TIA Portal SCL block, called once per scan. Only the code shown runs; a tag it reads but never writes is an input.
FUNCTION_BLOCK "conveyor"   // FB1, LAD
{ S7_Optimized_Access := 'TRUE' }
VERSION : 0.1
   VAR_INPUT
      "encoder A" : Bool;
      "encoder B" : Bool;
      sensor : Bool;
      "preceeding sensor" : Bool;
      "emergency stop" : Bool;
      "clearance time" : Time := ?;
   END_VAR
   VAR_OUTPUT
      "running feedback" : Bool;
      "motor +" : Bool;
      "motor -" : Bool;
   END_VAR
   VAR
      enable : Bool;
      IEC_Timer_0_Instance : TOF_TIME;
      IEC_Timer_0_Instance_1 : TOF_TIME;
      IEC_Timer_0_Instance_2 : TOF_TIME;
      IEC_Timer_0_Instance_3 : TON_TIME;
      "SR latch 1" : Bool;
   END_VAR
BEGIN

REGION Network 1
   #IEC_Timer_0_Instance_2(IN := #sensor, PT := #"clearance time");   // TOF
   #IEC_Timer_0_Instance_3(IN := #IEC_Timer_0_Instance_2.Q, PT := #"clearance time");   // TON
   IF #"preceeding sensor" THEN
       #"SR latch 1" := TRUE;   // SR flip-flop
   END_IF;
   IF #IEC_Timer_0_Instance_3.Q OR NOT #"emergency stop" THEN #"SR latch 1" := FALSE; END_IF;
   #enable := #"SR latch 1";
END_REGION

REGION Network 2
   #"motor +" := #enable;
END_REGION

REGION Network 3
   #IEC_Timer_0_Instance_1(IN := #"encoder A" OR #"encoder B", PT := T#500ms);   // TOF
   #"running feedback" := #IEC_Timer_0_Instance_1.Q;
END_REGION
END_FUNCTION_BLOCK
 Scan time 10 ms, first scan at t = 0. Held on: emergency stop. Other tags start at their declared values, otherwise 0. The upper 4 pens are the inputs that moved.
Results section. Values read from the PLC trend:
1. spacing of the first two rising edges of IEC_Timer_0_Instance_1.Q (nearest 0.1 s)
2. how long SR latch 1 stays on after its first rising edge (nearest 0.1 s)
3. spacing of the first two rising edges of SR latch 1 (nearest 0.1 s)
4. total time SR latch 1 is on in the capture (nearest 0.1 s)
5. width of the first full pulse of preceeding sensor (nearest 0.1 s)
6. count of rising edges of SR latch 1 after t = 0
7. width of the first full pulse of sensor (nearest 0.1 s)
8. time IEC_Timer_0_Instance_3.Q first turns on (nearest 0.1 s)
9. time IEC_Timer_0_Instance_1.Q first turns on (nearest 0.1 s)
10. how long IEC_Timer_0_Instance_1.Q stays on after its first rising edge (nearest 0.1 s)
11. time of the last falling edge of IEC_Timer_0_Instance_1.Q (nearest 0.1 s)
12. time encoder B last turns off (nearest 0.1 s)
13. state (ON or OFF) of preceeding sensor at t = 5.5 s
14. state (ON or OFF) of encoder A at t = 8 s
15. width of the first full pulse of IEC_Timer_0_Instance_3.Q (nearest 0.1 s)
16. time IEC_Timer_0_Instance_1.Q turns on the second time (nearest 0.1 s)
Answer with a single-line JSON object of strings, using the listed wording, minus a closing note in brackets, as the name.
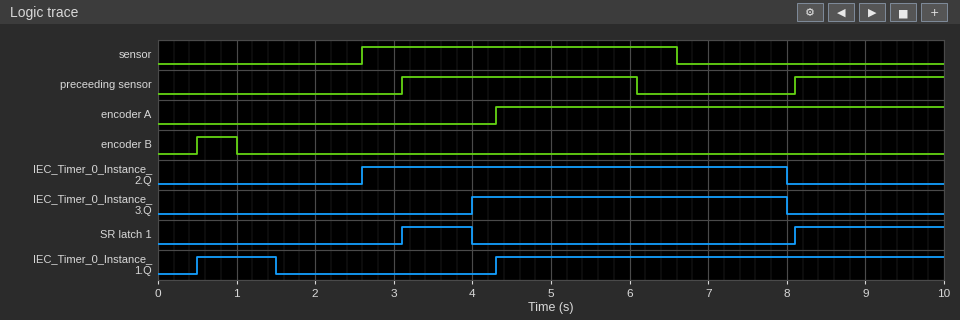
{"spacing of the first two rising edges of IEC_Timer_0_Instance_1.Q": "3.8 s", "how long SR latch 1 stays on after its first rising edge": "0.9 s", "spacing of the first two rising edges of SR latch 1": "5.0 s", "total time SR latch 1 is on in the capture": "2.8 s", "width of the first full pulse of preceeding sensor": "3.0 s", "count of rising edges of SR latch 1 after t = 0": "2", "width of the first full pulse of sensor": "4.0 s", "time IEC_Timer_0_Instance_3.Q first turns on": "4.0 s", "time IEC_Timer_0_Instance_1.Q first turns on": "0.5 s", "how long IEC_Timer_0_Instance_1.Q stays on after its first rising edge": "1.0 s", "time of the last falling edge of IEC_Timer_0_Instance_1.Q": "1.5 s", "time encoder B last turns off": "1.0 s", "state (ON or OFF) of preceeding sensor at t = 5.5 s": "ON", "state (ON or OFF) of encoder A at t = 8 s": "ON", "width of the first full pulse of IEC_Timer_0_Instance_3.Q": "4.0 s", "time IEC_Timer_0_Instance_1.Q turns on the second time": "4.3 s"}
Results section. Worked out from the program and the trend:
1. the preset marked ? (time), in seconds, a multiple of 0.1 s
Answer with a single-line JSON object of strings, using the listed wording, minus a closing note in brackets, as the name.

{"the preset marked ? (time), in seconds, a multiple of 0.1 s": "1.4 s"}
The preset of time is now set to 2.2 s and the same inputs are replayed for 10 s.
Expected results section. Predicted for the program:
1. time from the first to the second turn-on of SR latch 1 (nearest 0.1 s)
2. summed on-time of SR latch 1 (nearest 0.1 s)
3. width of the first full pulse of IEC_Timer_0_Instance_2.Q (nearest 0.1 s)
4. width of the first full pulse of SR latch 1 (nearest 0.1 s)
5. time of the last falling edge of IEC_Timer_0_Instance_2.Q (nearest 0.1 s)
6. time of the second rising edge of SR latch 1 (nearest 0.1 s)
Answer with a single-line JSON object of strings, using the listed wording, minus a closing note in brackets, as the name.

{"time from the first to the second turn-on of SR latch 1": "5.7 s", "summed on-time of SR latch 1": "2.9 s", "width of the first full pulse of IEC_Timer_0_Instance_2.Q": "6.2 s", "width of the first full pulse of SR latch 1": "1.7 s", "time of the last falling edge of IEC_Timer_0_Instance_2.Q": "8.8 s", "time of the second rising edge of SR latch 1": "8.8 s"}
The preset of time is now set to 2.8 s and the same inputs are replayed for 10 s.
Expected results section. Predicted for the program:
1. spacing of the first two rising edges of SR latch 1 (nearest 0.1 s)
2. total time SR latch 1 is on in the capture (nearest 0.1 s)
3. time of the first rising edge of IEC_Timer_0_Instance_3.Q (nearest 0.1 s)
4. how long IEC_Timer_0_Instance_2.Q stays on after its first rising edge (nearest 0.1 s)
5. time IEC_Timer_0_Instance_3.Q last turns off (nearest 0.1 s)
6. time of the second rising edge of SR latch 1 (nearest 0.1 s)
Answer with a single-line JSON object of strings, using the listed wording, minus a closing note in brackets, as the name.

{"spacing of the first two rising edges of SR latch 1": "6.3 s", "total time SR latch 1 is on in the capture": "2.9 s", "time of the first rising edge of IEC_Timer_0_Instance_3.Q": "5.4 s", "how long IEC_Timer_0_Instance_2.Q stays on after its first rising edge": "6.8 s", "time IEC_Timer_0_Instance_3.Q last turns off": "9.4 s", "time of the second rising edge of SR latch 1": "9.4 s"}
